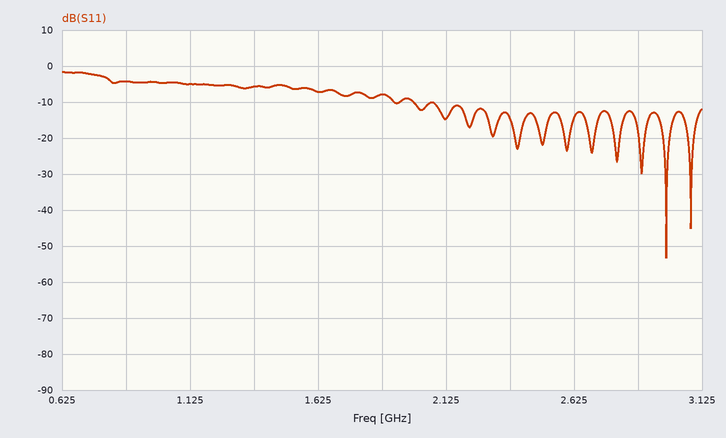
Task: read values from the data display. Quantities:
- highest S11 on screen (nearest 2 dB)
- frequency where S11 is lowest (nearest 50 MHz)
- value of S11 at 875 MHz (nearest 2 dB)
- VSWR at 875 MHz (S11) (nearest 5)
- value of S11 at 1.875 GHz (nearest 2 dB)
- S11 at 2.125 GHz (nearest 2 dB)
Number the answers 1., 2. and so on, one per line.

1. -2 dB
2. 3.00 GHz
3. -4 dB
4. 5
5. -8 dB
6. -14 dB
